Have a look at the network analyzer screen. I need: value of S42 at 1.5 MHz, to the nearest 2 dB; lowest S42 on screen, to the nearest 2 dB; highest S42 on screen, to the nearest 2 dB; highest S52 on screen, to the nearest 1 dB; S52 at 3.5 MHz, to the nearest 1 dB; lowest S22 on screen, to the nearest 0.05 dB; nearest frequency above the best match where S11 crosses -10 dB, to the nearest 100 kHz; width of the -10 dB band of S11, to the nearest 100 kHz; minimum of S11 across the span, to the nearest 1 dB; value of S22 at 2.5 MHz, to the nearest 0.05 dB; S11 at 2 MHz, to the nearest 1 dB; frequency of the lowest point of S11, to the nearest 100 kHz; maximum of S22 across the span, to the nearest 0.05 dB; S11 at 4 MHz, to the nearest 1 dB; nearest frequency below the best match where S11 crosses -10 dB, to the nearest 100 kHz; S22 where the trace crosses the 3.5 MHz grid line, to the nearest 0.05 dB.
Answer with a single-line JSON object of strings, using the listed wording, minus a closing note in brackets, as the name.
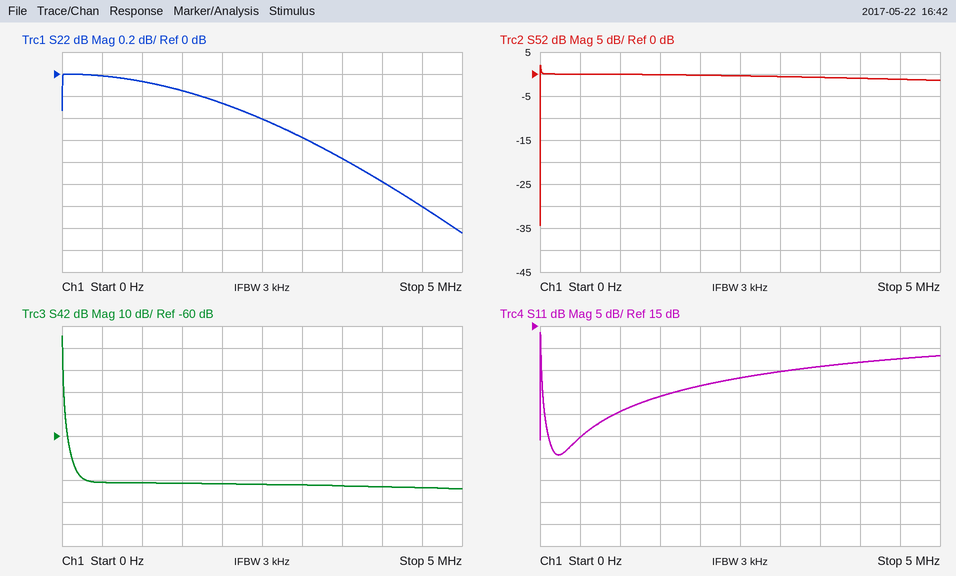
{"value of S42 at 1.5 MHz, to the nearest 2 dB": "-82 dB", "lowest S42 on screen, to the nearest 2 dB": "-84 dB", "highest S42 on screen, to the nearest 2 dB": "-14 dB", "highest S52 on screen, to the nearest 1 dB": "2 dB", "S52 at 3.5 MHz, to the nearest 1 dB": "-1 dB", "lowest S22 on screen, to the nearest 0.05 dB": "-1.45 dB", "nearest frequency above the best match where S11 crosses -10 dB, to the nearest 100 kHz": "500 kHz", "width of the -10 dB band of S11, to the nearest 100 kHz": "400 kHz", "minimum of S11 across the span, to the nearest 1 dB": "-14 dB", "value of S22 at 2.5 MHz, to the nearest 0.05 dB": "-0.40 dB", "S11 at 2 MHz, to the nearest 1 dB": "1 dB", "frequency of the lowest point of S11, to the nearest 100 kHz": "200 kHz", "maximum of S22 across the span, to the nearest 0.05 dB": "0.00 dB", "S11 at 4 MHz, to the nearest 1 dB": "7 dB", "nearest frequency below the best match where S11 crosses -10 dB, to the nearest 100 kHz": "100 kHz", "S22 where the trace crosses the 3.5 MHz grid line, to the nearest 0.05 dB": "-0.75 dB"}
